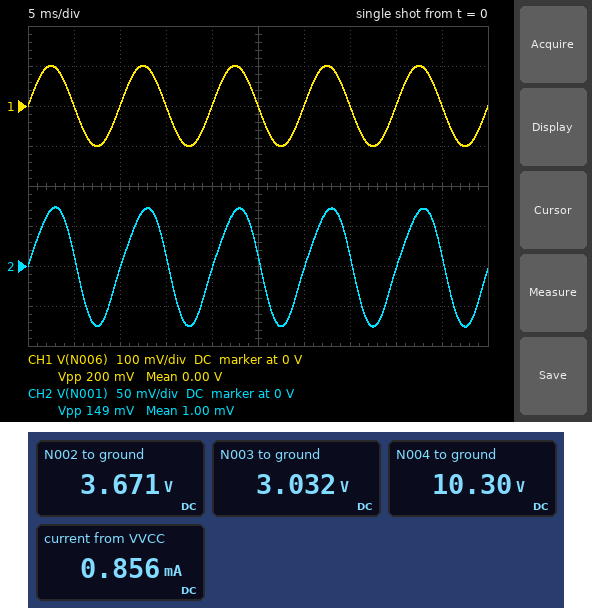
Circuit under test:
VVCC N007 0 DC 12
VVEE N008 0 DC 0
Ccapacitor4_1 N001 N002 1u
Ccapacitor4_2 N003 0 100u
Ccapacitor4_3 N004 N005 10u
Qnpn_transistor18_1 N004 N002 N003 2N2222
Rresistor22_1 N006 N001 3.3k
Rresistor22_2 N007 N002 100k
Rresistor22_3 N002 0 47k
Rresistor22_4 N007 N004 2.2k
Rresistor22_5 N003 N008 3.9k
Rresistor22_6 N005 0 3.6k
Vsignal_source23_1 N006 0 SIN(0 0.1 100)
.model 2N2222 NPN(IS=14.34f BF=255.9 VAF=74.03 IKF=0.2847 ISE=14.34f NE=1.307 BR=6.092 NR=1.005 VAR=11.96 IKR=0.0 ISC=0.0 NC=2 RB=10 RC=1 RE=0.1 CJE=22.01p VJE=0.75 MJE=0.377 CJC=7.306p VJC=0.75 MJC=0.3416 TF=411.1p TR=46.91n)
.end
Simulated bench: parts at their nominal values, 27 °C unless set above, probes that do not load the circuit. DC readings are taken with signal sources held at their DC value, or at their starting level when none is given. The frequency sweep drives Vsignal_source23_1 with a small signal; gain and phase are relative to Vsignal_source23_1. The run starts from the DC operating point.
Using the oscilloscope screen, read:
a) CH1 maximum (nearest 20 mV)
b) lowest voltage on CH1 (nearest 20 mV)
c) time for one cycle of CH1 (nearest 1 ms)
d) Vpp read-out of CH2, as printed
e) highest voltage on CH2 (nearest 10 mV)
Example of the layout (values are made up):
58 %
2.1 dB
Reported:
100 mV
-100 mV
10 ms
149 mV
70 mV
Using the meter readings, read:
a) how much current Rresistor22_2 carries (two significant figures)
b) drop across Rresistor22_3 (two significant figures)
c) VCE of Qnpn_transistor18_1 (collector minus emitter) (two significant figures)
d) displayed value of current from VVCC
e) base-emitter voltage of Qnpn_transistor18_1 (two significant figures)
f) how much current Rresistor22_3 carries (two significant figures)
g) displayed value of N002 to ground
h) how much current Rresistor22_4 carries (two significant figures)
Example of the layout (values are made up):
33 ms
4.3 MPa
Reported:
83 µA
3.7 V
7.3 V
0.856 mA
640 mV
78 µA
3.671 V
770 µA
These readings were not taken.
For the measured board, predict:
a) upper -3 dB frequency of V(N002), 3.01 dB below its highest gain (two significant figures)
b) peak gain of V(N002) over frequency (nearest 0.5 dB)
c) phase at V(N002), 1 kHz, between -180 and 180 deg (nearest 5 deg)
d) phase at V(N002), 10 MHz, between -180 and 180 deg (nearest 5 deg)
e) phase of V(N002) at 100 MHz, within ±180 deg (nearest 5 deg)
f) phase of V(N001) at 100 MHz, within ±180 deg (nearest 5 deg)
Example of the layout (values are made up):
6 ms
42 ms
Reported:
440 kHz
-4.5 dB
0 deg
-70 deg
-40 deg
-40 deg
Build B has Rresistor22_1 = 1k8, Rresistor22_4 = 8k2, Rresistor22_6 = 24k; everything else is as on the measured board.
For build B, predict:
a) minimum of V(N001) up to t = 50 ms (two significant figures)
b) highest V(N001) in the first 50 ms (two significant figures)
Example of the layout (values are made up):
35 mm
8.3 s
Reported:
-84 mV
78 mV
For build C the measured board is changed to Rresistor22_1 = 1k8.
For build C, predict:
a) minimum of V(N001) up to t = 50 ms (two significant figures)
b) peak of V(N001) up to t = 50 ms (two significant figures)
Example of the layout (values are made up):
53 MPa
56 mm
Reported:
-86 mV
84 mV
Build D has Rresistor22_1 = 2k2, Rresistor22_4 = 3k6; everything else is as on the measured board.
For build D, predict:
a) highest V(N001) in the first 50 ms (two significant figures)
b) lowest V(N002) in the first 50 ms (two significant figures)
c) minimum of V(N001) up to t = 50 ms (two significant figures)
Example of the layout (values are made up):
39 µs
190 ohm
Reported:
81 mV
3.6 V
-83 mV
